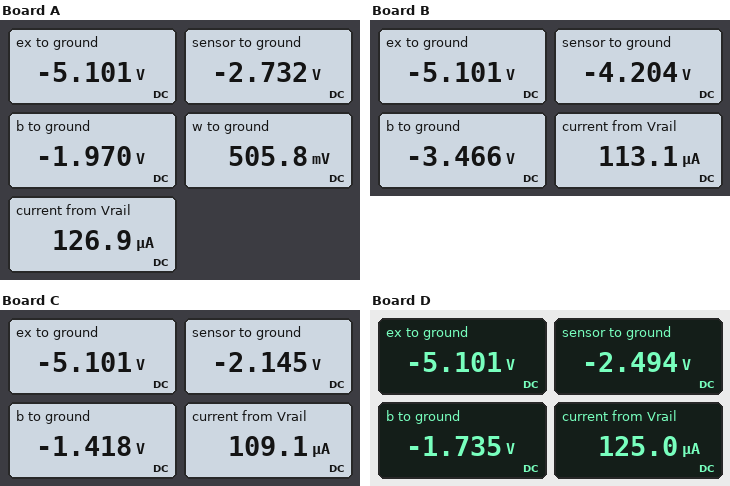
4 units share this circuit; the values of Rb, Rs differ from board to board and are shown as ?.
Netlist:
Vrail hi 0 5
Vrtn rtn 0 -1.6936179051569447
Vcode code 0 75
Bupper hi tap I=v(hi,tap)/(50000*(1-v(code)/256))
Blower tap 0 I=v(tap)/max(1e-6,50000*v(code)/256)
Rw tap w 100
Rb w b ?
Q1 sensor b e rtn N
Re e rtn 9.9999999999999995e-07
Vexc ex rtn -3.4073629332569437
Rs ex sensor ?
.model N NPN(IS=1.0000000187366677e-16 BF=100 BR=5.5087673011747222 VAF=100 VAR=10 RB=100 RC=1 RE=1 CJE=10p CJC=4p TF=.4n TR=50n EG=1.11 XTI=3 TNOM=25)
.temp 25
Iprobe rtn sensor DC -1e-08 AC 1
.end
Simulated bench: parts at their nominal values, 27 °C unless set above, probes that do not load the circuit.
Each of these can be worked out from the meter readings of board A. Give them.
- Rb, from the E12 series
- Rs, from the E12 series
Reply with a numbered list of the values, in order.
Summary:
1. 27 kΩ
2. 3.9 kΩ
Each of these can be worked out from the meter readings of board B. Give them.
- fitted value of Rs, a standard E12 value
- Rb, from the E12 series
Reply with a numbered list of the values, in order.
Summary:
1. 2.7 kΩ
2. 100 kΩ
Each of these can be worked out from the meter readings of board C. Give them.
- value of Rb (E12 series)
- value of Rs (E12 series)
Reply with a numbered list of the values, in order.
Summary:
1. 82 kΩ
2. 15 kΩ
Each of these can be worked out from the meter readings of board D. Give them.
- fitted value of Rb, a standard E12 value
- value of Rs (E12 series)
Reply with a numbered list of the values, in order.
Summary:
1. 27 kΩ
2. 4.7 kΩ
